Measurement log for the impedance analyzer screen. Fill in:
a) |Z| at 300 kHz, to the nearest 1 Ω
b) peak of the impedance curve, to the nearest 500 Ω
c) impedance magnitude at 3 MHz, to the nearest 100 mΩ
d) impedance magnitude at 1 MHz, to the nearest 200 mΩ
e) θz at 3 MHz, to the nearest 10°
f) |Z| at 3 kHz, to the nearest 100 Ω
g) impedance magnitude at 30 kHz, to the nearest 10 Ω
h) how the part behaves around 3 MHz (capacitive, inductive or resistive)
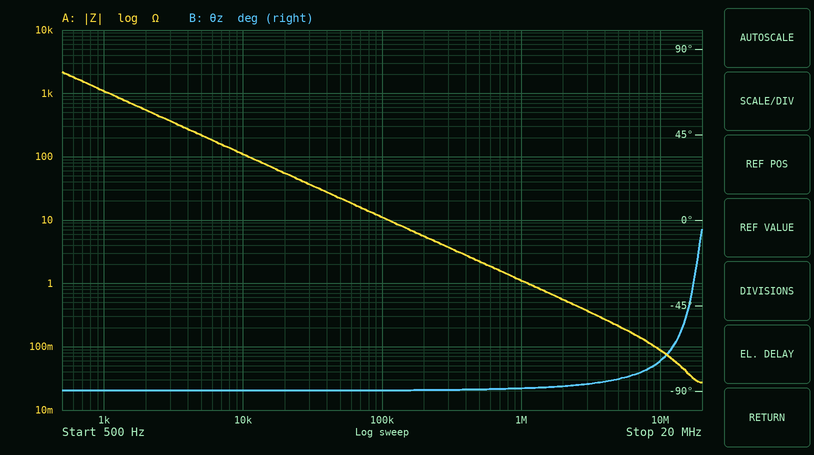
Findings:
4 Ω
2.0 kΩ
400 mΩ
1.2 Ω
-90°
400 Ω
40 Ω
capacitive
